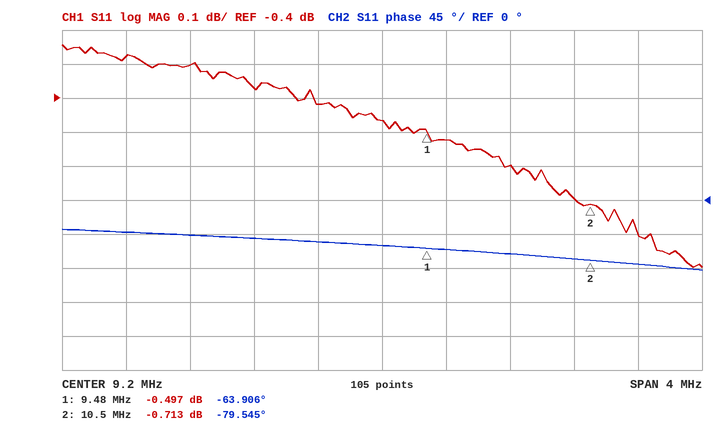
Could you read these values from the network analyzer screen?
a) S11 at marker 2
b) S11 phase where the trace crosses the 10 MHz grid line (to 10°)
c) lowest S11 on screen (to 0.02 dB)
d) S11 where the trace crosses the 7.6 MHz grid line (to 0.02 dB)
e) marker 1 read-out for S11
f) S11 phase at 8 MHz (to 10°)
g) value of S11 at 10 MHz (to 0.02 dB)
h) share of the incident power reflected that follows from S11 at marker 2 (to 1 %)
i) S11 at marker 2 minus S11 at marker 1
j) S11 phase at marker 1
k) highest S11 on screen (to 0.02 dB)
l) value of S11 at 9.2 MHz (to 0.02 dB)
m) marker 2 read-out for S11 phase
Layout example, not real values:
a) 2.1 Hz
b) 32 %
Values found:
a) -0.713 dB
b) -70°
c) -0.90 dB
d) -0.28 dB
e) -0.497 dB
f) -50°
g) -0.60 dB
h) 85 %
i) -0.216 dB
j) -63.906°
k) -0.24 dB
l) -0.46 dB
m) -79.545°
